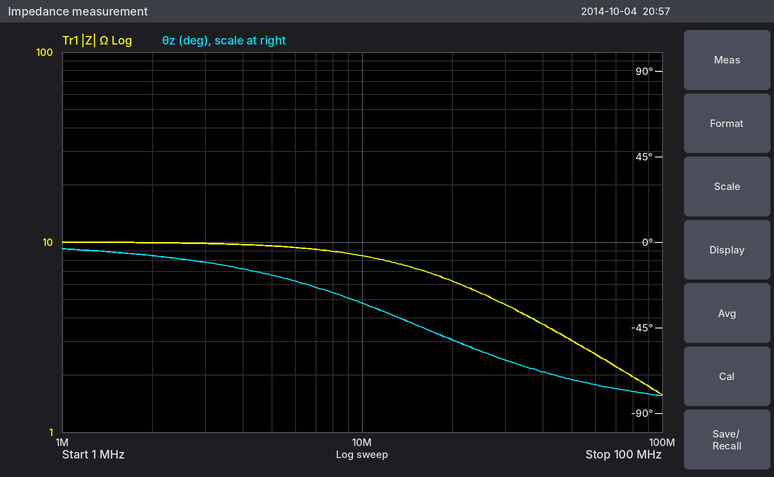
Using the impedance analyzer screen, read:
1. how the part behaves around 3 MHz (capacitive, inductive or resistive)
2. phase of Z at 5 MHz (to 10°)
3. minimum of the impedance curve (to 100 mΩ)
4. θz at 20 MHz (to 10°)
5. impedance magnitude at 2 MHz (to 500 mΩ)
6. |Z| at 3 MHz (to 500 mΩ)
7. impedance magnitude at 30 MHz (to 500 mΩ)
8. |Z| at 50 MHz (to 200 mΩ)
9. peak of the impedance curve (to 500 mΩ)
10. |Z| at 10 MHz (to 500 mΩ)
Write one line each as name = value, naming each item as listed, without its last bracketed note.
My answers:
how the part behaves around 3 MHz = resistive
phase of Z at 5 MHz = -20°
minimum of the impedance curve = 1.6 Ω
θz at 20 MHz = -50°
impedance magnitude at 2 MHz = 10.0 Ω
|Z| at 3 MHz = 10.0 Ω
impedance magnitude at 30 MHz = 4.5 Ω
|Z| at 50 MHz = 3.0 Ω
peak of the impedance curve = 10.0 Ω
|Z| at 10 MHz = 8.5 Ω
